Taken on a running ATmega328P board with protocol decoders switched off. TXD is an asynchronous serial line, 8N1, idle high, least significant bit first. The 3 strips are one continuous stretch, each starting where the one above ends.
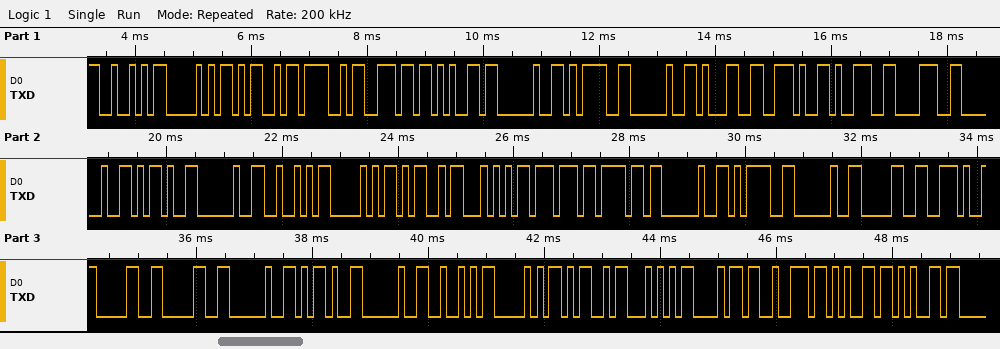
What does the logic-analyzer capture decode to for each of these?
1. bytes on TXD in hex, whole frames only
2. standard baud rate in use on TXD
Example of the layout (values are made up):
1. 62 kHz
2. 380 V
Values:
1. 52 50 4D 4F 6E 65 20 3D 20 31 2E 39 38 20 2D 20 52 50 4D 54 77 6F 20 3D 20 30 2E 30 30 20 2D 20 52 50 4D 54 68 72 65 65
2. 9600 baud
